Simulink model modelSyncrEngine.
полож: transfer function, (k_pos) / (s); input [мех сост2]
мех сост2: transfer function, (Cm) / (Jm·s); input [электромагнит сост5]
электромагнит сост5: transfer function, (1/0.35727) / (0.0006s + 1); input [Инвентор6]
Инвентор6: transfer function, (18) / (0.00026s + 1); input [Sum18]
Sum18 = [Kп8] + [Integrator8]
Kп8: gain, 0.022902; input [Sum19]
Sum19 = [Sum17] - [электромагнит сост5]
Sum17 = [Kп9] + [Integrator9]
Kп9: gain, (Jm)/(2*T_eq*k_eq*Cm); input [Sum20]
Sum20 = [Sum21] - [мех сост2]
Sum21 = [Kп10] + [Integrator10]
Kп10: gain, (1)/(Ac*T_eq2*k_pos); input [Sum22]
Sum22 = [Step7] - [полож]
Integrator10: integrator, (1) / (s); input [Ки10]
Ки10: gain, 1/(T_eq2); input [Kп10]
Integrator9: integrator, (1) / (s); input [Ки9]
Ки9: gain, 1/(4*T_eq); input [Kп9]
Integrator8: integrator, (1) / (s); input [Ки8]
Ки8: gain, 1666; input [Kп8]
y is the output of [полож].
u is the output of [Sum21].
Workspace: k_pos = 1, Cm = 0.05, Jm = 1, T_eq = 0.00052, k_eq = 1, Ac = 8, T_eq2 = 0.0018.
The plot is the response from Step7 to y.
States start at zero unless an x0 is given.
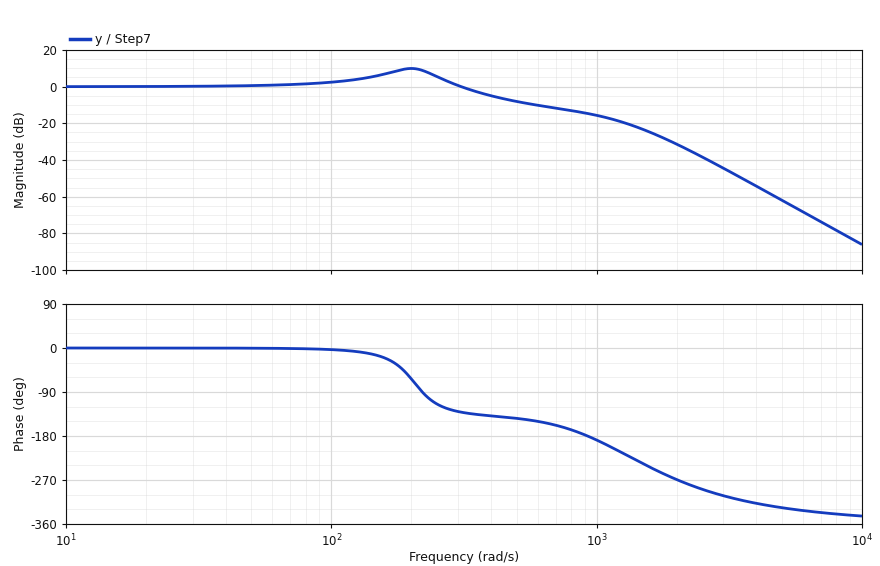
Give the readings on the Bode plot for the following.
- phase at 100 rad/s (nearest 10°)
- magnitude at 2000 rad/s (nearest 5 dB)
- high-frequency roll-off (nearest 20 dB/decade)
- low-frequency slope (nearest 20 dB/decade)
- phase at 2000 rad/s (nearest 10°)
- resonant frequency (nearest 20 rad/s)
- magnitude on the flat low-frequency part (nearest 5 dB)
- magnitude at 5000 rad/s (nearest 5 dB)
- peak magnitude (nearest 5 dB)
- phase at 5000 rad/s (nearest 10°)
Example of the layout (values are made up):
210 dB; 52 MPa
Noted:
0°; -30 dB; -80 dB/decade; 0 dB/decade; -270°; 200 rad/s; 0 dB; -60 dB; 10 dB; -330°
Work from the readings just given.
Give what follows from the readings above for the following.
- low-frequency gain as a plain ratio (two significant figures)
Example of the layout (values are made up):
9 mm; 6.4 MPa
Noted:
1.0
